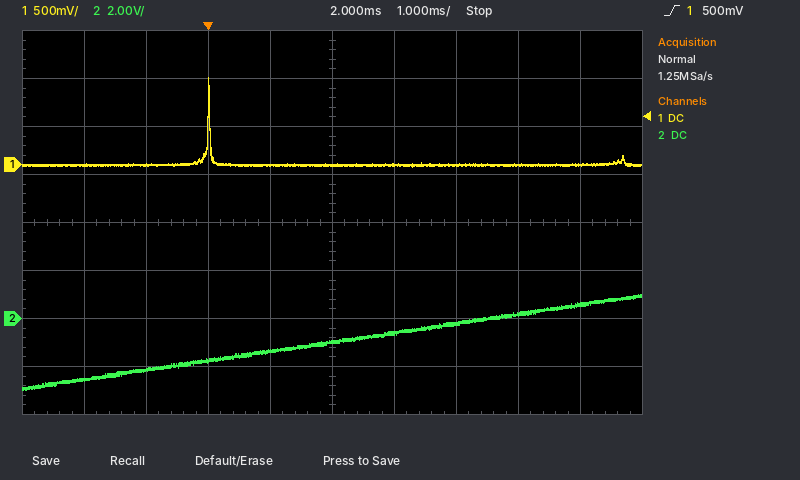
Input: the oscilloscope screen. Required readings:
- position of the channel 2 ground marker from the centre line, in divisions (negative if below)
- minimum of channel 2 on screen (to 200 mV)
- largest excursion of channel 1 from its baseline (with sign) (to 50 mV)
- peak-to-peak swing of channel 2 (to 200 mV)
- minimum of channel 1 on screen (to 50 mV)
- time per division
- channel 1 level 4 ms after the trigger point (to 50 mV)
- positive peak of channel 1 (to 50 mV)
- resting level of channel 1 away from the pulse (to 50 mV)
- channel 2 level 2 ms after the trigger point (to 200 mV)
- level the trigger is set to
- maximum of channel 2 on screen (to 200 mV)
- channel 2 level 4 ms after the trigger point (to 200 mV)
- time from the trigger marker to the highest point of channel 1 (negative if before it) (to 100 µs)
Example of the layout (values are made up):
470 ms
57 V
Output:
-2.0 div
-3.0 V
+900 mV
4.0 V
0 mV
1 ms
0 mV
900 mV
0 mV
-1.0 V
500 mV
1.0 V
-200 mV
0.0 ms
